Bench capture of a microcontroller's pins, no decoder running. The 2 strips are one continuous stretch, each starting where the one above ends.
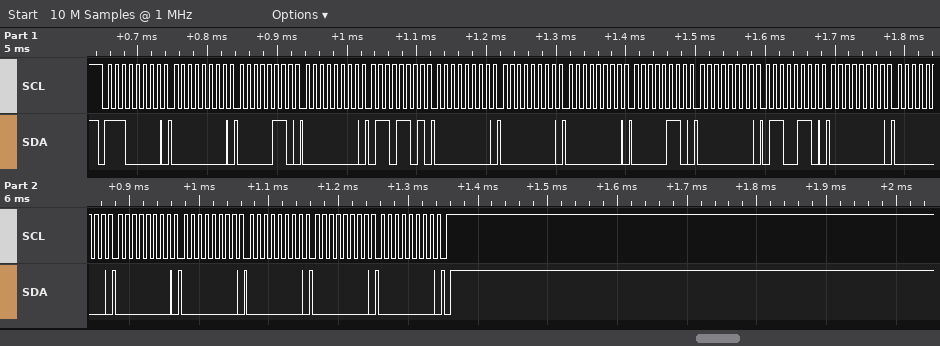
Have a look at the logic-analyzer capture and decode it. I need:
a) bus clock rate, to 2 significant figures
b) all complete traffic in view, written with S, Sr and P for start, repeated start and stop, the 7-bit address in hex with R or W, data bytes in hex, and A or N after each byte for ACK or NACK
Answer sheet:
100 kHz
S 70W A 00 A 06 A 00 A 6D A 00 A 00 A 00 A 06 A 00 A 66 A 00 A 00 A 00 A 00 A 00 A 00 A 00 A P
